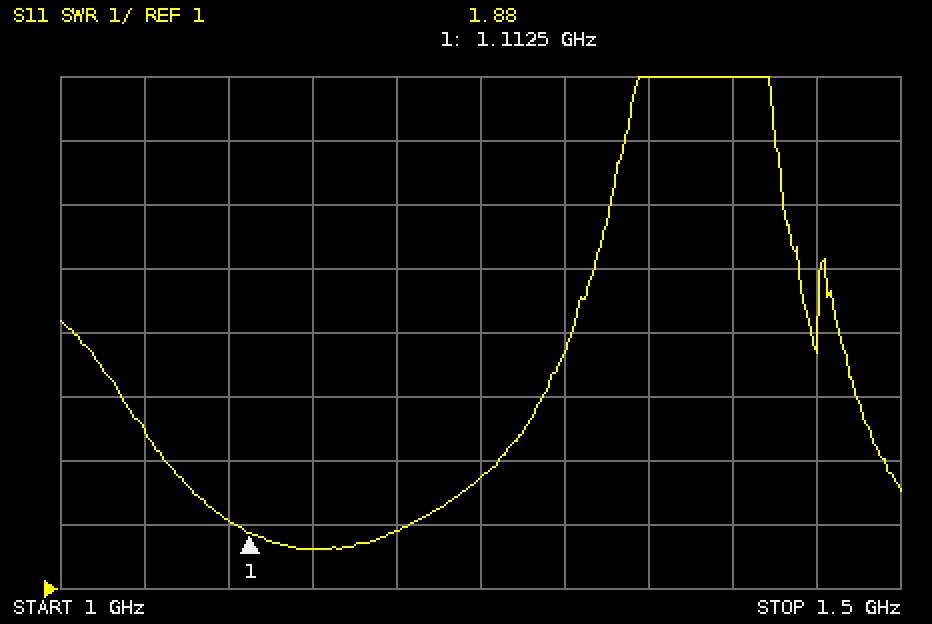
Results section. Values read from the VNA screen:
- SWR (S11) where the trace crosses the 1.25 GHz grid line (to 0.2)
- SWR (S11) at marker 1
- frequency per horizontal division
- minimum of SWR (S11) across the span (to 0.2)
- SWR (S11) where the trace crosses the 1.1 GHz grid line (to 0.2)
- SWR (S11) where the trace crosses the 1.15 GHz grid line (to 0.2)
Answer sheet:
2.8
1.88
50 MHz
1.6
2.0
1.6
